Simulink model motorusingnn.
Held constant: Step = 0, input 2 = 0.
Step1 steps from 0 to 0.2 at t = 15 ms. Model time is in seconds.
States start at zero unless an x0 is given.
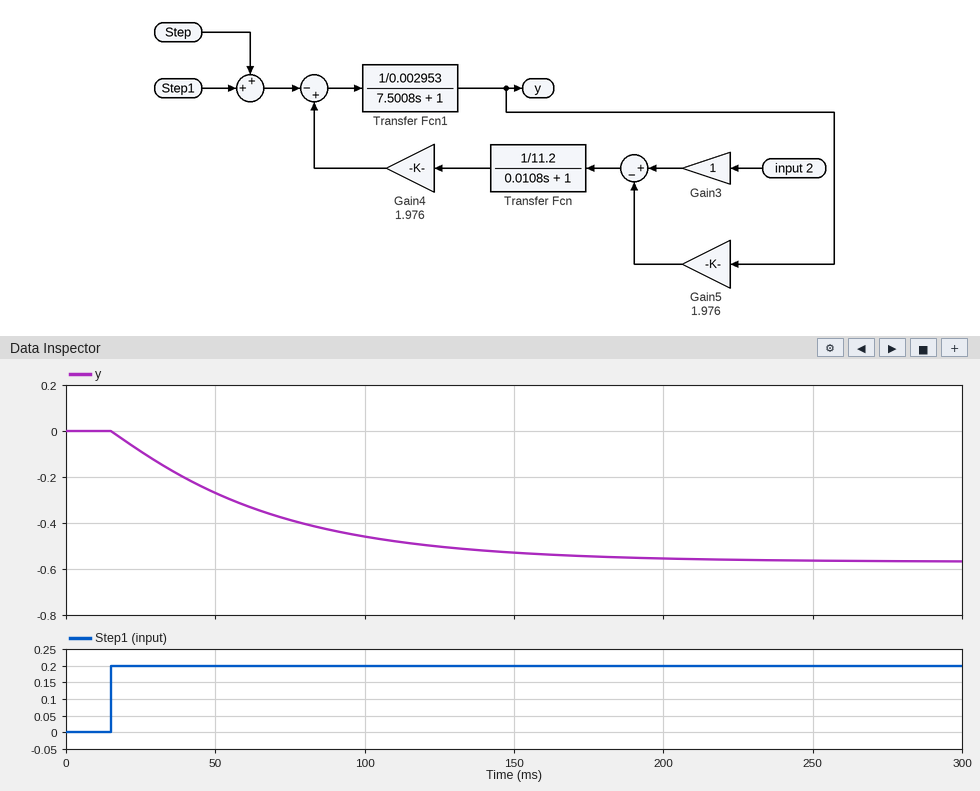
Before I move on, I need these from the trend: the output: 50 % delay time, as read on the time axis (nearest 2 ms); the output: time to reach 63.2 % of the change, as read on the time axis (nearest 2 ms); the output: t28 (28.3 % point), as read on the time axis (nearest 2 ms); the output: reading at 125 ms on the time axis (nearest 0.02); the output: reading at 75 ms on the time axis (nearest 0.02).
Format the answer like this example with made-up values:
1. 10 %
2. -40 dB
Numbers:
1. 52 ms
2. 68 ms
3. 34 ms
4. -0.50
5. -0.38
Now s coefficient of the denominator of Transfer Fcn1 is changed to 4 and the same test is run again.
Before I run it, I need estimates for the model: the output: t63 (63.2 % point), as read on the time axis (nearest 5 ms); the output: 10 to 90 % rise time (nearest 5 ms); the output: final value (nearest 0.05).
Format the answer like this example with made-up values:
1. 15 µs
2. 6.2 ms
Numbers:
1. 40 ms
2. 45 ms
3. -0.55
